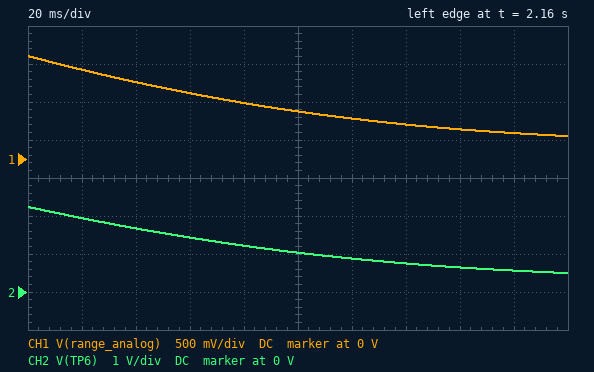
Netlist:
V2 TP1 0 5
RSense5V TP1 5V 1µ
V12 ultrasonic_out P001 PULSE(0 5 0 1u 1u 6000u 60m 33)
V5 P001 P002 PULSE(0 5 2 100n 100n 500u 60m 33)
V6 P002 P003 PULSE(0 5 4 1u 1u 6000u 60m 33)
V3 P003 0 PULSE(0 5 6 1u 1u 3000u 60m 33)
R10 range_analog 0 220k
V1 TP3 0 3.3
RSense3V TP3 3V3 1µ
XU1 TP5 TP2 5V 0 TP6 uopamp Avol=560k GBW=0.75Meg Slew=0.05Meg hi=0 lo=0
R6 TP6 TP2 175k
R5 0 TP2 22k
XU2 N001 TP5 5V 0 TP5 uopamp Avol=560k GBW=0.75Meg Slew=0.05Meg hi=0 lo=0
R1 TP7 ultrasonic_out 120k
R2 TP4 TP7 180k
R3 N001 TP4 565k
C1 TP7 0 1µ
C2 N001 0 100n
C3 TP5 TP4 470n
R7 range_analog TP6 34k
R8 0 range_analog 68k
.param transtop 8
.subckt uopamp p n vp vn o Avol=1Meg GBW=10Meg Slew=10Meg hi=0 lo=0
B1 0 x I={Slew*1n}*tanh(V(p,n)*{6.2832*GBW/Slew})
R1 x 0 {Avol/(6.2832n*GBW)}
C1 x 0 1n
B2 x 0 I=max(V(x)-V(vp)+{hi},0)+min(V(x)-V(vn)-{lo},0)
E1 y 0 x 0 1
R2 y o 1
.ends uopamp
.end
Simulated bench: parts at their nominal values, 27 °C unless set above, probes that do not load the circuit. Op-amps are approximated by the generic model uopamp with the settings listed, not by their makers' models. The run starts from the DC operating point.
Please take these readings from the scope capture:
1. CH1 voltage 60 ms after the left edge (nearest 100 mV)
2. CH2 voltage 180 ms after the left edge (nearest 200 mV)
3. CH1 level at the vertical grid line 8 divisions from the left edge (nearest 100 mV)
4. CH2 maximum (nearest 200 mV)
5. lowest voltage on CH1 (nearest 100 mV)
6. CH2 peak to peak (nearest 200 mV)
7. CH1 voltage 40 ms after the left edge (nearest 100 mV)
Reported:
900 mV
600 mV
400 mV
2.2 V
300 mV
1.8 V
1.0 V
